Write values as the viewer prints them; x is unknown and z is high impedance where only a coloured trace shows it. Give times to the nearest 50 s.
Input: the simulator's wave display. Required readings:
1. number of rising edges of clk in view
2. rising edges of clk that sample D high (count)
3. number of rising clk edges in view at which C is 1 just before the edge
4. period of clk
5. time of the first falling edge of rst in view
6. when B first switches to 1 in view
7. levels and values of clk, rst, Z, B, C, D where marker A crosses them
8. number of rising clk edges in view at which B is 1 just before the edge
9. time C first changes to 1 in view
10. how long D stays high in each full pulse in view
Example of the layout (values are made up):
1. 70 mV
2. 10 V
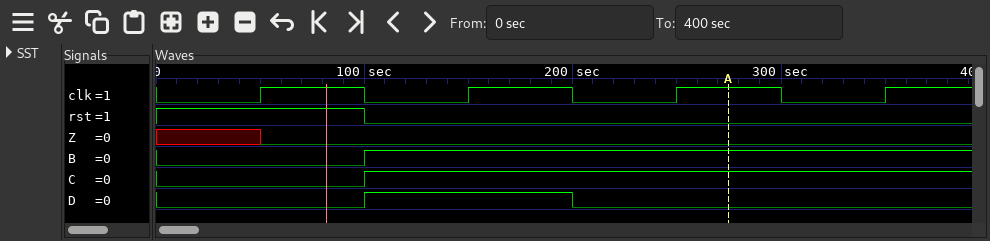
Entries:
1. 4
2. 1
3. 3
4. 100 s
5. 100 s
6. 100 s
7. clk=1, rst=0, Z=0, B=1, C=1, D=0
8. 3
9. 100 s
10. 100 s
